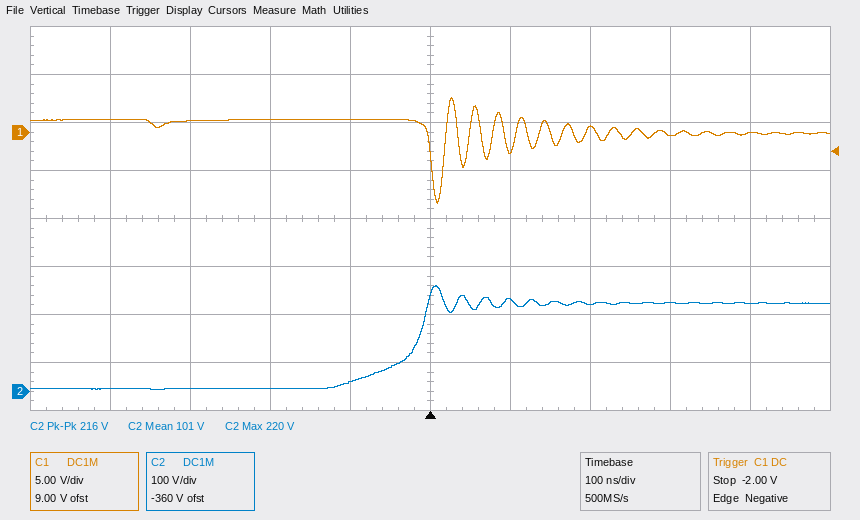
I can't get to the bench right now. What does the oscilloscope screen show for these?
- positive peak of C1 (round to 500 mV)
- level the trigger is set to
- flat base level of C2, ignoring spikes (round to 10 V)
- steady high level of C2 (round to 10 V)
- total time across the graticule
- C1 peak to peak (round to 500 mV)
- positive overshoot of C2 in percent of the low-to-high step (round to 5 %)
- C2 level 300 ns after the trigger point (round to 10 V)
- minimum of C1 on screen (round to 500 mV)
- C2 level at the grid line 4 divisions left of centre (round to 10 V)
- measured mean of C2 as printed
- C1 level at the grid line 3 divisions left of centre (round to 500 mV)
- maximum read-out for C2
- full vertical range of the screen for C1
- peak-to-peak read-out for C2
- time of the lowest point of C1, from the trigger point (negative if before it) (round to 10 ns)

3.5 V
-2.00 V
10 V
180 V
1 µs
11.0 V
20 %
180 V
-7.5 V
10 V
101 V
1.0 V
220 V
40 V
216 V
+10 ns
